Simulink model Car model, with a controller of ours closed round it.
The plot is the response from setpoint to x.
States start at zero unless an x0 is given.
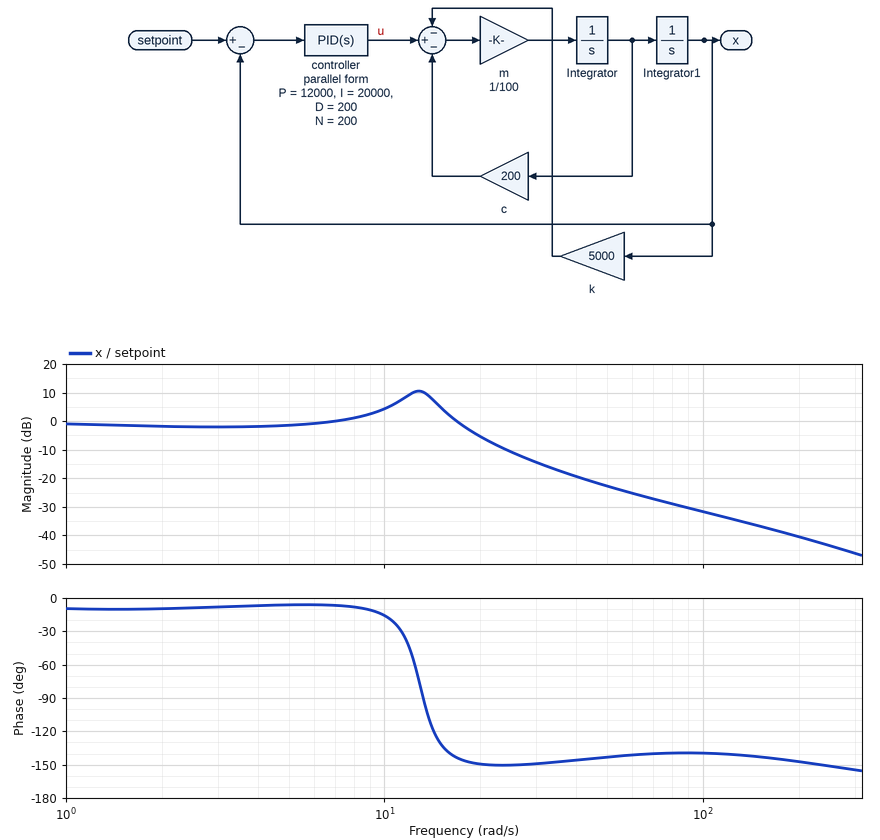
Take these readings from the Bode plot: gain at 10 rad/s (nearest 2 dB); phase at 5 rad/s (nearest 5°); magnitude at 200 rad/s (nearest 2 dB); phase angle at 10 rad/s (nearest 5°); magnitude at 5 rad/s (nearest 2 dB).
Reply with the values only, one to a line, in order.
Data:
4 dB
-5°
-40 dB
-15°
-2 dB
